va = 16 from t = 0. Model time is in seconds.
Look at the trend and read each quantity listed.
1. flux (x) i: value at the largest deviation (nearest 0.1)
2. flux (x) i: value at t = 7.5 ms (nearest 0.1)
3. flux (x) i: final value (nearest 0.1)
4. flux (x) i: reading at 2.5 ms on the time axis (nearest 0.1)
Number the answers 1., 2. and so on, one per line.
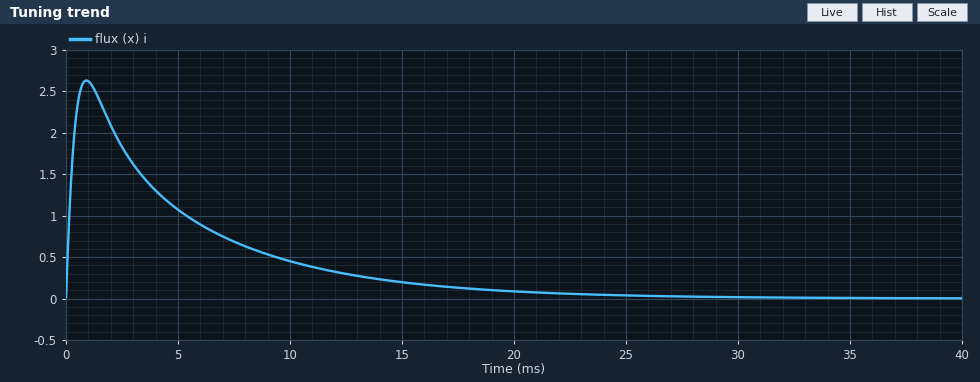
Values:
1. 2.6
2. 0.7
3. 0.0
4. 1.8
